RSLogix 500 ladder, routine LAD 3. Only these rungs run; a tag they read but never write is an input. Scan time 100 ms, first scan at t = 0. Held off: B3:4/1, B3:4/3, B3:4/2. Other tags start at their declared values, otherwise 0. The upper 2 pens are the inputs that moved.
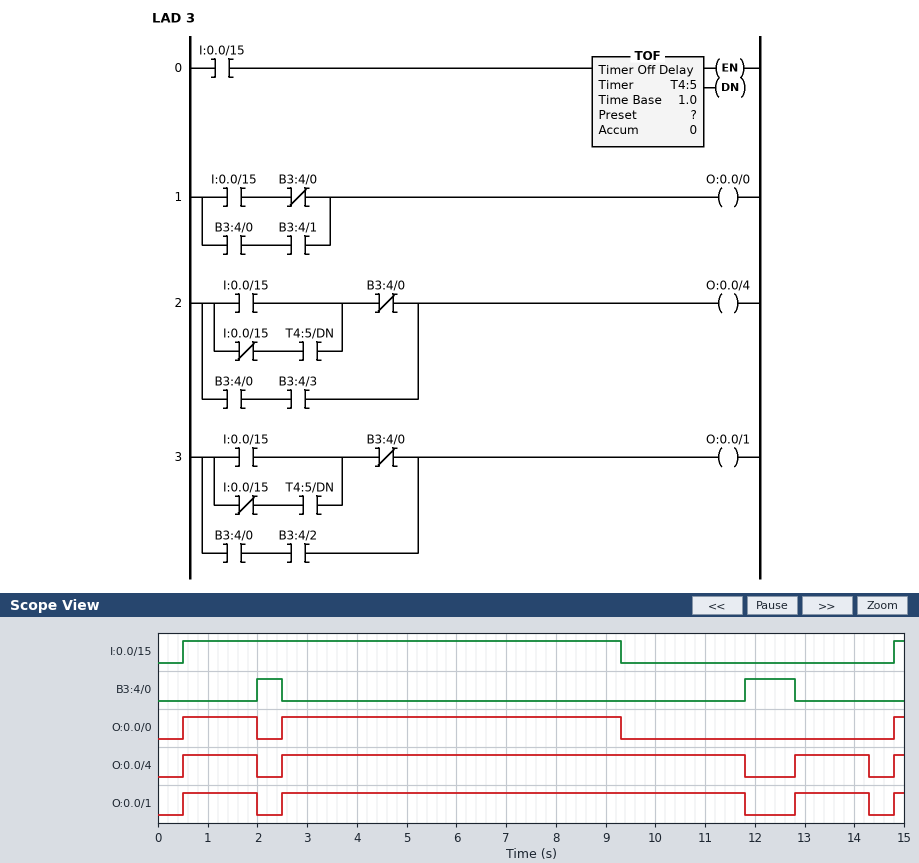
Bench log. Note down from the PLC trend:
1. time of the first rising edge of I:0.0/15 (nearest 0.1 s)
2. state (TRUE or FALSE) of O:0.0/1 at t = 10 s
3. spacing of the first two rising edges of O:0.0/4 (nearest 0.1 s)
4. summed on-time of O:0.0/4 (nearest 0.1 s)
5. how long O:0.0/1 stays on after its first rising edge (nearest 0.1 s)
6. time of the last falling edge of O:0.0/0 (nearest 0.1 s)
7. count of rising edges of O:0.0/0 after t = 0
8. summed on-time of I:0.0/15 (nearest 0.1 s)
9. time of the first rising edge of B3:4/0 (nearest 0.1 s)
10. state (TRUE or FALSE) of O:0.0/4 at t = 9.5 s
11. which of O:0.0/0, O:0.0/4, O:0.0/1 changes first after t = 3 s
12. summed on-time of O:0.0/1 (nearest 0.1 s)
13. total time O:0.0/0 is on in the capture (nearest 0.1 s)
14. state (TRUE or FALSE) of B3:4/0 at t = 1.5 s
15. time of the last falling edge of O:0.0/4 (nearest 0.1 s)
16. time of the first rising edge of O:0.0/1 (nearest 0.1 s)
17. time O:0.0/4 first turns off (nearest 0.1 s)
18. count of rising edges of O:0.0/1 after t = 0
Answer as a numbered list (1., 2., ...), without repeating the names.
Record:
1. 0.5 s
2. TRUE
3. 2.0 s
4. 12.5 s
5. 1.5 s
6. 9.3 s
7. 3
8. 9.0 s
9. 2.0 s
10. TRUE
11. O:0.0/0
12. 12.5 s
13. 8.5 s
14. FALSE
15. 14.3 s
16. 0.5 s
17. 2.0 s
18. 4
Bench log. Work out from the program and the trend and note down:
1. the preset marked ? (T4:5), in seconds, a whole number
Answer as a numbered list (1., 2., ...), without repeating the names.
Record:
1. 5 s
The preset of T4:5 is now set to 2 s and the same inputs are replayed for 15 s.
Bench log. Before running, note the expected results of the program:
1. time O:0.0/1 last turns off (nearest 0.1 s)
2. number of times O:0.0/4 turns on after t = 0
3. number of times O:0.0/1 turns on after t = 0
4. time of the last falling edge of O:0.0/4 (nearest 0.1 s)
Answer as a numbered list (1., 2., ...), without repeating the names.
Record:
1. 11.3 s
2. 3
3. 3
4. 11.3 s
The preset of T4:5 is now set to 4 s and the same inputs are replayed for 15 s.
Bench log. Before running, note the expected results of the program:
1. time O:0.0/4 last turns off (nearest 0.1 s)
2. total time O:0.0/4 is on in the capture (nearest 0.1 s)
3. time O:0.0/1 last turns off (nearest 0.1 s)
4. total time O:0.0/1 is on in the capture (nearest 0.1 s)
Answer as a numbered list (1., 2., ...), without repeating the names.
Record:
1. 13.3 s
2. 11.5 s
3. 13.3 s
4. 11.5 s
